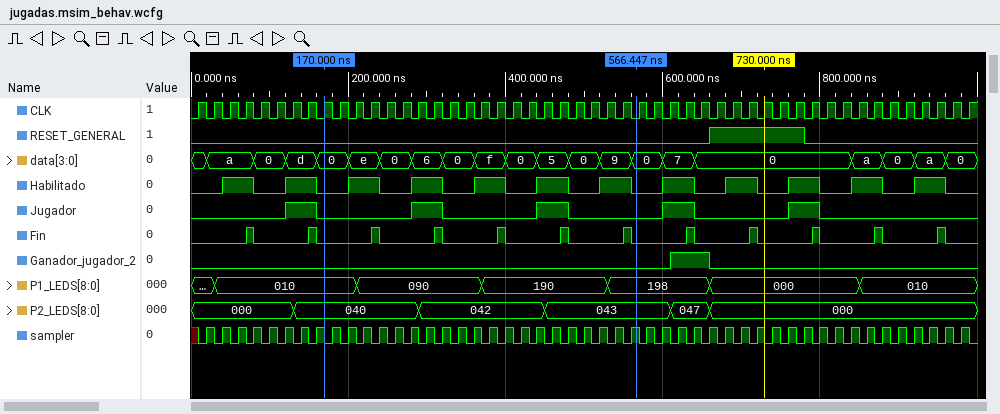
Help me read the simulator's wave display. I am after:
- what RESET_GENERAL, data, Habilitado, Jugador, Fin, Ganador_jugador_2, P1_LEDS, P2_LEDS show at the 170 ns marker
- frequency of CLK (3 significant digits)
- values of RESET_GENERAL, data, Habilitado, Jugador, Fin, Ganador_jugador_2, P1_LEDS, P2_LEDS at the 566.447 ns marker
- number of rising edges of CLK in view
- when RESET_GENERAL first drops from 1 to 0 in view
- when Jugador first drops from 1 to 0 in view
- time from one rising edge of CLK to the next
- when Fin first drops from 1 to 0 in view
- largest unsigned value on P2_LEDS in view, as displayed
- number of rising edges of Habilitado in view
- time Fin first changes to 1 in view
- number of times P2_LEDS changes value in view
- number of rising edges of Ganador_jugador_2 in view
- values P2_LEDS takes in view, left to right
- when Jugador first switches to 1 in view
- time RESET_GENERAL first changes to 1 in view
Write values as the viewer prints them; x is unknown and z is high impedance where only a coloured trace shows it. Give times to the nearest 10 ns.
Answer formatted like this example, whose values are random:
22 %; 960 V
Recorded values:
RESET_GENERAL=0, data=0, Habilitado=0, Jugador=0, Fin=0, Ganador_jugador_2=0, P1_LEDS=010, P2_LEDS=040; 50.0 MHz; RESET_GENERAL=0, data=0, Habilitado=0, Jugador=0, Fin=0, Ganador_jugador_2=0, P1_LEDS=198, P2_LEDS=043; 50; 780 ns; 160 ns; 20 ns; 80 ns; 047; 12; 70 ns; 5; 1; 000, 040, 042, 043, 047, 000; 120 ns; 660 ns
